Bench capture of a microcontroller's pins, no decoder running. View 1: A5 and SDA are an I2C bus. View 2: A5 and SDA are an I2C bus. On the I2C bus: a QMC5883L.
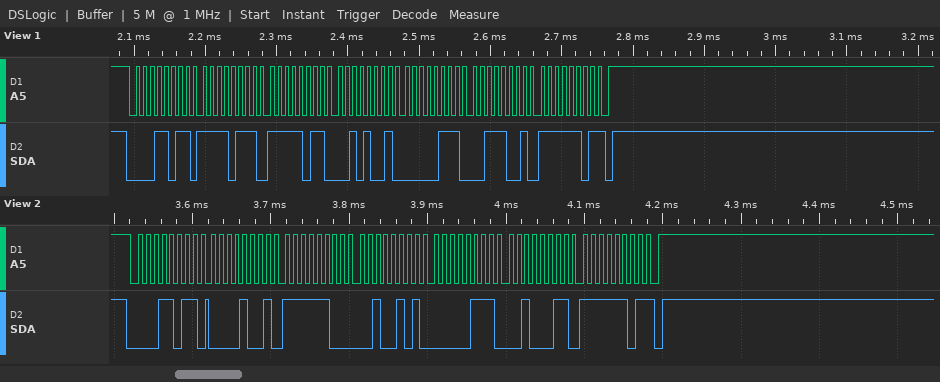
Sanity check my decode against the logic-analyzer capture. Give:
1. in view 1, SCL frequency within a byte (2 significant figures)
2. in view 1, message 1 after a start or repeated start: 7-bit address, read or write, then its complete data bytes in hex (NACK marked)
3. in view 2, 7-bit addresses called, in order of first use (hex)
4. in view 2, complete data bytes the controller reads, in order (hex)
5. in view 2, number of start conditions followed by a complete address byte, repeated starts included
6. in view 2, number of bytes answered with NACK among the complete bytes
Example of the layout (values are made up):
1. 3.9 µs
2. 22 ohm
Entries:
1. 100 kHz
2. 0x0D read: F7 FB 29 07 39 FD NACK
3. 0x0D
4. 09 FC 25 07 23 FD
5. 1
6. 1
